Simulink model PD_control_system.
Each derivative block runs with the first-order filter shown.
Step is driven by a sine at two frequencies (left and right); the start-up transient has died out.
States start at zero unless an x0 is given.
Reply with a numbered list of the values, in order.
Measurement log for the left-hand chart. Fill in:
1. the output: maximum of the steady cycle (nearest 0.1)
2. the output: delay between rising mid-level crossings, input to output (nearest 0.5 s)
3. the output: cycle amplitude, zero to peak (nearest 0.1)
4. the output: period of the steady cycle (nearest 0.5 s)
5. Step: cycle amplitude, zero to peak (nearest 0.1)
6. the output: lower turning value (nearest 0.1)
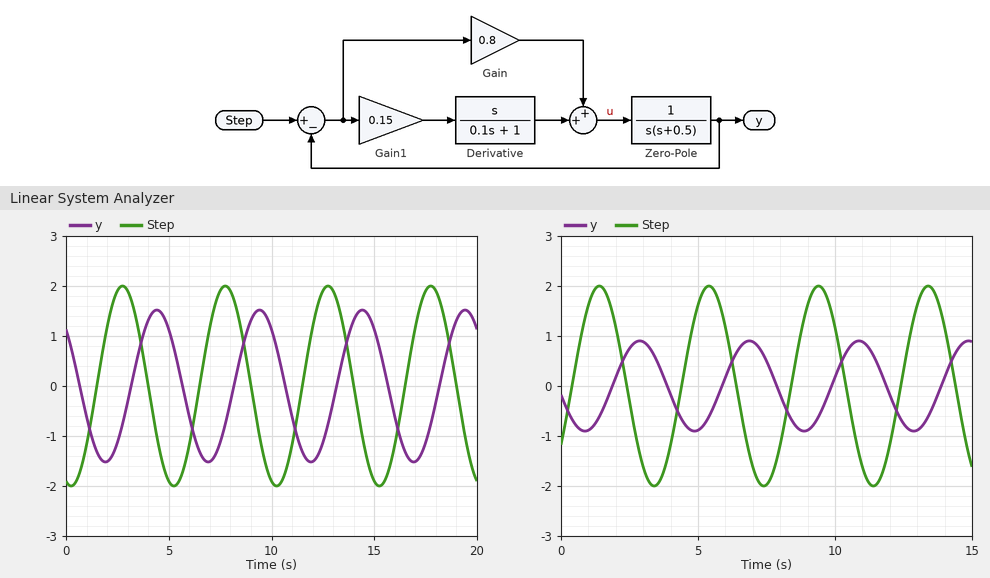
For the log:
1. 1.5
2. 1.5 s
3. 1.5
4. 5.0 s
5. 2.0
6. -1.5
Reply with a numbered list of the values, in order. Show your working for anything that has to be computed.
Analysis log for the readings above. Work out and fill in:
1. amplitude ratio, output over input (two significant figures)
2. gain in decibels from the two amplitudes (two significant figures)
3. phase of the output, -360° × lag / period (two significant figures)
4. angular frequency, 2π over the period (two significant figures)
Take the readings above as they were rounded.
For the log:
1. 1.5 / 2 = 0.75
2. 20 log10(1.5 / 2) = -2.5 dB
3. -360 × 1.5 / 5 = -110°
4. 2π / 5 = 1.3 rad/s
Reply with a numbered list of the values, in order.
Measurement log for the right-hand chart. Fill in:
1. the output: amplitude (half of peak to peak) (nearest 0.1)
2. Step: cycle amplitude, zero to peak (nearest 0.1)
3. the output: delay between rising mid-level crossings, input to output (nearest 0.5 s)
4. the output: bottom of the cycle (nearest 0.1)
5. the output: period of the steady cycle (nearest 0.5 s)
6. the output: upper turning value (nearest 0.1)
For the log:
1. 0.9
2. 2.0
3. 1.5 s
4. -0.9
5. 4.0 s
6. 0.9
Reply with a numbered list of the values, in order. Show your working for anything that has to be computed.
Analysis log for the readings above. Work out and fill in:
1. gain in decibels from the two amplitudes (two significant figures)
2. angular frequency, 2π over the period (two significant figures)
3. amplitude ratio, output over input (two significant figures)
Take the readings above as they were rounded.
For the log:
1. 20 log10(0.9 / 2) = -6.9 dB
2. 2π / 4 = 1.6 rad/s
3. 0.9 / 2 = 0.45
